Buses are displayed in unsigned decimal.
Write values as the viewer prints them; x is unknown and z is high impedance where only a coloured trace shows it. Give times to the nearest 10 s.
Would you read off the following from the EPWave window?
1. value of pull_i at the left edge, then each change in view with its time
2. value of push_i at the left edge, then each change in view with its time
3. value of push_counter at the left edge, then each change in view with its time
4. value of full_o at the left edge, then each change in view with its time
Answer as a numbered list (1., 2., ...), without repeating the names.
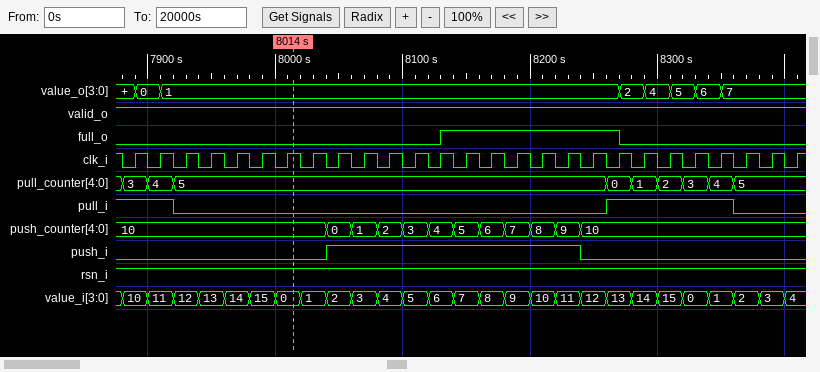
1. 1, 0 at 7920 s, 1 at 8260 s, 0 at 8360 s
2. 0, 1 at 8040 s, 0 at 8240 s
3. 10, 0 at 8040 s, 1 at 8060 s, 2 at 8080 s, 3 at 8100 s, 4 at 8120 s, 5 at 8140 s, 6 at 8160 s, 7 at 8180 s, 8 at 8200 s, 9 at 8220 s, 10 at 8240 s
4. 0, 1 at 8130 s, 0 at 8270 s
